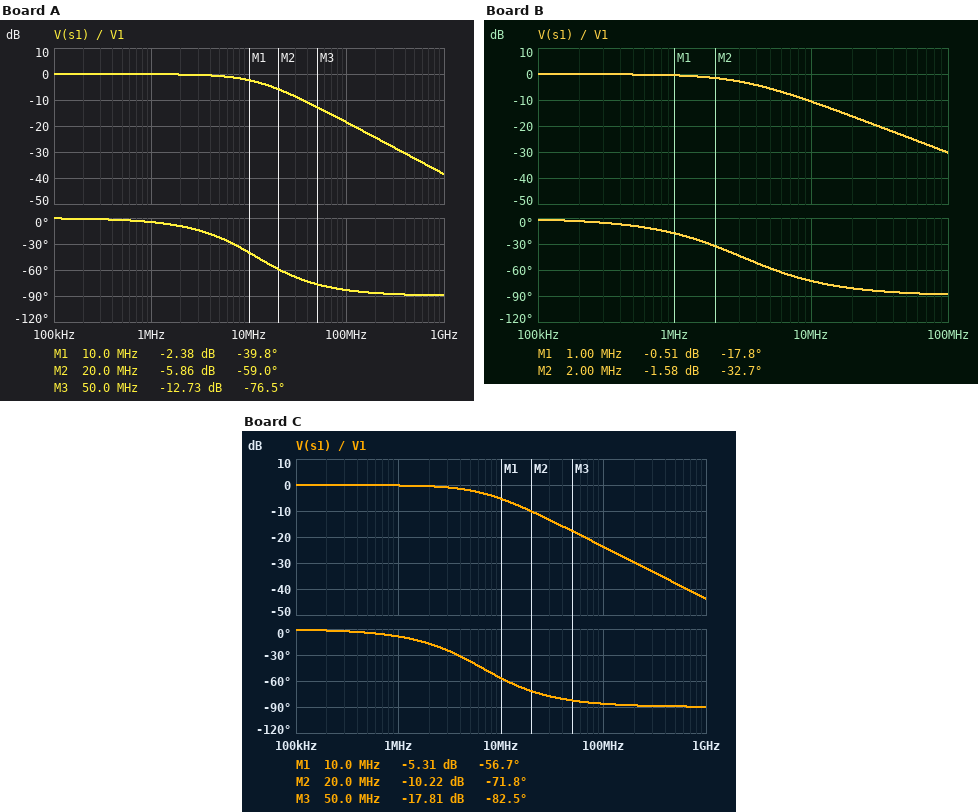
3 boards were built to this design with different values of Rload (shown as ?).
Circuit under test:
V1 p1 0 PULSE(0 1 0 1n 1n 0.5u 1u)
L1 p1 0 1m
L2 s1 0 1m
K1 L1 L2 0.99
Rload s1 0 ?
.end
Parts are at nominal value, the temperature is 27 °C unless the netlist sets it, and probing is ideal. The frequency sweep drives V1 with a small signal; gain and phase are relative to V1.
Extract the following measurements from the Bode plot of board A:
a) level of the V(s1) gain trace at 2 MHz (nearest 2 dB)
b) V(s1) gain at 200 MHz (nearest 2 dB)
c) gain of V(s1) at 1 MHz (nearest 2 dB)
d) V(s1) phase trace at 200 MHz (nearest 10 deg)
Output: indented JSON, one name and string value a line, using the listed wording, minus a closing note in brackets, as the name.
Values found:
{
  "level of the V(s1) gain trace at 2 MHz": "0 dB",
  "V(s1) gain at 200 MHz": "-24 dB",
  "gain of V(s1) at 1 MHz": "0 dB",
  "V(s1) phase trace at 200 MHz": "-90 deg"
}
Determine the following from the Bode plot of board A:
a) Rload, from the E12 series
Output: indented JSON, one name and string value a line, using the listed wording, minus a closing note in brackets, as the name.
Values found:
{
  "Rload, from the E12 series": "1.5 kΩ"
}
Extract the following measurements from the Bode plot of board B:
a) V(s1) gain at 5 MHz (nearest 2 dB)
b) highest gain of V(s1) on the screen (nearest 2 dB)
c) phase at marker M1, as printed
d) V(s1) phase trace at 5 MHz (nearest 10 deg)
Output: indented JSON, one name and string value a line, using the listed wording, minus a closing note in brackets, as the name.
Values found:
{
  "V(s1) gain at 5 MHz": "-6 dB",
  "highest gain of V(s1) on the screen": "0 dB",
  "phase at marker M1, as printed": "-17.8 deg",
  "V(s1) phase trace at 5 MHz": "-60 deg"
}
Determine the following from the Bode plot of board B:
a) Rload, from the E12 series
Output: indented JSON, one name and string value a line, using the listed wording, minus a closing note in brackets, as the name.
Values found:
{
  "Rload, from the E12 series": "390 Ω"
}
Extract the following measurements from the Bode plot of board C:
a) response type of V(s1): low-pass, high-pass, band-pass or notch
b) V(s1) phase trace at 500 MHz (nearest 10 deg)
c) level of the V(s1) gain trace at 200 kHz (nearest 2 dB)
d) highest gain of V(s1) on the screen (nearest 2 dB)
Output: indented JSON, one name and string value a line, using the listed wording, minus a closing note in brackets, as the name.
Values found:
{
  "response type of V(s1): low-pass, high-pass, band-pass or notch": "low-pass",
  "V(s1) phase trace at 500 MHz": "-90 deg",
  "level of the V(s1) gain trace at 200 kHz": "0 dB",
  "highest gain of V(s1) on the screen": "0 dB"
}
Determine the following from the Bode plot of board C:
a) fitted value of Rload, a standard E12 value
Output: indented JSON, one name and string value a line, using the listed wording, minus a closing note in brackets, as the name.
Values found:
{
  "fitted value of Rload, a standard E12 value": "820 Ω"
}
